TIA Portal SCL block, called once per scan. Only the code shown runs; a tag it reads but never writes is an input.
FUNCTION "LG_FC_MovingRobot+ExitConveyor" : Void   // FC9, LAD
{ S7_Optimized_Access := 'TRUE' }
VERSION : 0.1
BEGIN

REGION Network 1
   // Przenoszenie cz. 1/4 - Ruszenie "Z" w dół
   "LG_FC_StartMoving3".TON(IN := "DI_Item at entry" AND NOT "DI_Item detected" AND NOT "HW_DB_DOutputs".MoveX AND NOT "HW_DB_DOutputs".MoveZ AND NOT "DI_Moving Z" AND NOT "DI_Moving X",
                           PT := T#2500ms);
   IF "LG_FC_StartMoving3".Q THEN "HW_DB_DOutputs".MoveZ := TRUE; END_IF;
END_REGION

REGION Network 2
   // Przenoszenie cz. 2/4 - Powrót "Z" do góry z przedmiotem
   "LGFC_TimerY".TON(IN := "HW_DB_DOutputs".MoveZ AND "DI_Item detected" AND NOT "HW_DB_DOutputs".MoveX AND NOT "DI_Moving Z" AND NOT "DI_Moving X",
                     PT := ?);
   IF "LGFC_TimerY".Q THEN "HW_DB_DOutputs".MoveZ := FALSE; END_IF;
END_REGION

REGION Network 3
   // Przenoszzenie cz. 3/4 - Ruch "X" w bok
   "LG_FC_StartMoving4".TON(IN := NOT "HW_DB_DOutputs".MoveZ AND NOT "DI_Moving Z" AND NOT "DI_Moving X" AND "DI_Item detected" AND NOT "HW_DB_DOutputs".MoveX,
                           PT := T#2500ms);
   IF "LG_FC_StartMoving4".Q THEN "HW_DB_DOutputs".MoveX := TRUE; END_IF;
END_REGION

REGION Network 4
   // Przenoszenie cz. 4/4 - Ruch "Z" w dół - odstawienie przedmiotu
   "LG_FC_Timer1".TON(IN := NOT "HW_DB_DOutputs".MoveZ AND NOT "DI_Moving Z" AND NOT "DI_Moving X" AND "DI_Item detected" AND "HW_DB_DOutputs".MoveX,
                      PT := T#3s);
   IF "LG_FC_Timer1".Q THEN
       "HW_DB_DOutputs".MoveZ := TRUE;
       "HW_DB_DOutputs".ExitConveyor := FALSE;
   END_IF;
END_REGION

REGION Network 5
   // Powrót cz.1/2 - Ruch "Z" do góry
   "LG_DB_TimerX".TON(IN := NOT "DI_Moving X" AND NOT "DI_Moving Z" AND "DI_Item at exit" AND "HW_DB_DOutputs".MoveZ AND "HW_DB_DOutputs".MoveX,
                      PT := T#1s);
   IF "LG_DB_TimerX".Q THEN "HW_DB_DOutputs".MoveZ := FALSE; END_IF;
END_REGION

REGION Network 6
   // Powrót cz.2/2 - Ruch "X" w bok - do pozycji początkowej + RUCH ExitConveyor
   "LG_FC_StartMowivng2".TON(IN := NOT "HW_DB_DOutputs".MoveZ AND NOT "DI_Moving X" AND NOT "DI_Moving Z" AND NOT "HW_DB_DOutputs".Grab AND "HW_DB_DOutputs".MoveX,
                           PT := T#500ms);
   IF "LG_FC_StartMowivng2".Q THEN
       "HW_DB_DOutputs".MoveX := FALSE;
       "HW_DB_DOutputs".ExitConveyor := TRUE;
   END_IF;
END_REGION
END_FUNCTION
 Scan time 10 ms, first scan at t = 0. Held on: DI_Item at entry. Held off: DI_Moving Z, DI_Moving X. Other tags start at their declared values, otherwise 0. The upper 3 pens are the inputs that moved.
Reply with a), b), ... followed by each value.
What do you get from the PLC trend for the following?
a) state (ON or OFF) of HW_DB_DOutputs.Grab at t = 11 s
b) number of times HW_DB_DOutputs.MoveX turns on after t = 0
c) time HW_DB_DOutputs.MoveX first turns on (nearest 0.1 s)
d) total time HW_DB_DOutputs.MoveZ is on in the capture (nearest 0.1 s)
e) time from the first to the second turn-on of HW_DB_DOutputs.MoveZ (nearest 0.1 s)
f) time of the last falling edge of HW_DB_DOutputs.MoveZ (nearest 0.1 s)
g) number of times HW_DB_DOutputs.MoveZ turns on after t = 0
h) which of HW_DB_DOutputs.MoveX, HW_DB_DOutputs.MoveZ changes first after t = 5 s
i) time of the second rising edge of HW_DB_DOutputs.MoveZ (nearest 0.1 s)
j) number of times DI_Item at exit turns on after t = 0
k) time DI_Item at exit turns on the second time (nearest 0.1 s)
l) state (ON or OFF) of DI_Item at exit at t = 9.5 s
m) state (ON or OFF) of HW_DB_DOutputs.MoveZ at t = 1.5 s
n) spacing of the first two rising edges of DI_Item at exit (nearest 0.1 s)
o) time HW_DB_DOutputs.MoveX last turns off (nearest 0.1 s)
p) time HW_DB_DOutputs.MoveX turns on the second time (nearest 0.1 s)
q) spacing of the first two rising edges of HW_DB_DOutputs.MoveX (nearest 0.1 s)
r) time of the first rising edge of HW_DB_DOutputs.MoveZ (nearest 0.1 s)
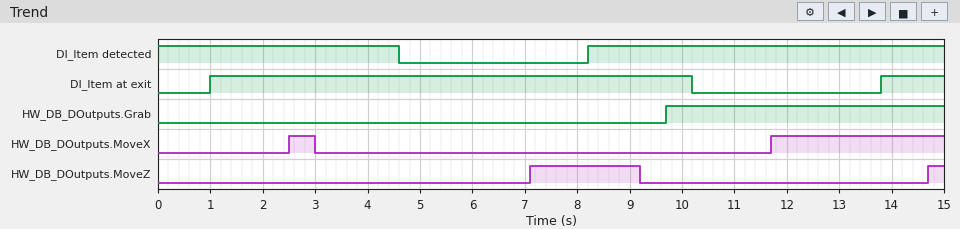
a) ON
b) 2
c) 2.5 s
d) 2.4 s
e) 7.6 s
f) 9.2 s
g) 2
h) HW_DB_DOutputs.MoveZ
i) 14.7 s
j) 2
k) 13.8 s
l) ON
m) OFF
n) 12.8 s
o) 3.0 s
p) 11.7 s
q) 9.2 s
r) 7.1 s
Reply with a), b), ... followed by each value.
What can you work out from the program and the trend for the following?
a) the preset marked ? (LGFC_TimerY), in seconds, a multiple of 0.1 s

a) 1.0 s
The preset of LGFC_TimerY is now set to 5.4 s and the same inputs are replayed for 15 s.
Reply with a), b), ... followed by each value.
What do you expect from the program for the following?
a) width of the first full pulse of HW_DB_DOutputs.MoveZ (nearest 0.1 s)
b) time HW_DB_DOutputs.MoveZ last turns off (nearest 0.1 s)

a) 6.5 s
b) 13.6 s
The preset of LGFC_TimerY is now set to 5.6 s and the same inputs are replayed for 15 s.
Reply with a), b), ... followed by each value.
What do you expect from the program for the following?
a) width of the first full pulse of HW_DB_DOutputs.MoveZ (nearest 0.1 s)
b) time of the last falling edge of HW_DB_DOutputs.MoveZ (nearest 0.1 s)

a) 6.7 s
b) 13.8 s
